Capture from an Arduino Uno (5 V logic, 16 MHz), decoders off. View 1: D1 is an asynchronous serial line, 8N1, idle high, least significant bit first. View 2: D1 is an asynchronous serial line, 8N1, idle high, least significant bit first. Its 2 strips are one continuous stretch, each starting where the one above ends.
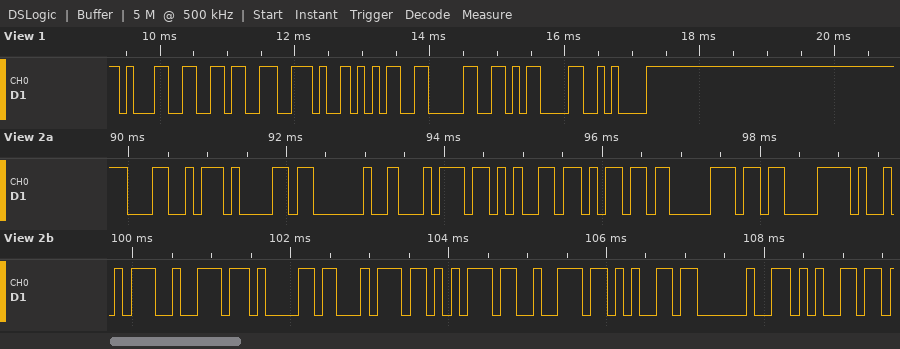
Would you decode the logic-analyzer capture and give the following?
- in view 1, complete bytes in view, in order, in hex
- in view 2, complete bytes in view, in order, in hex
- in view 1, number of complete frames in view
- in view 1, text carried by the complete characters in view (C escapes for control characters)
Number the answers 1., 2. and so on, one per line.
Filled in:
1. 31 36 2E 35 30 0D 0A
2. 4C 61 20 74 65 6D 70 C3 A9 72 61 74 75 72 65 20 65
3. 7
4. "16.50\r\n"
